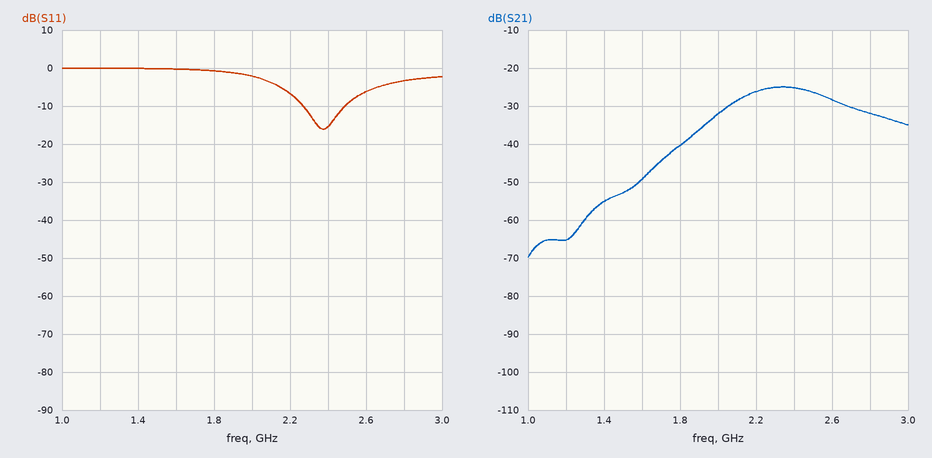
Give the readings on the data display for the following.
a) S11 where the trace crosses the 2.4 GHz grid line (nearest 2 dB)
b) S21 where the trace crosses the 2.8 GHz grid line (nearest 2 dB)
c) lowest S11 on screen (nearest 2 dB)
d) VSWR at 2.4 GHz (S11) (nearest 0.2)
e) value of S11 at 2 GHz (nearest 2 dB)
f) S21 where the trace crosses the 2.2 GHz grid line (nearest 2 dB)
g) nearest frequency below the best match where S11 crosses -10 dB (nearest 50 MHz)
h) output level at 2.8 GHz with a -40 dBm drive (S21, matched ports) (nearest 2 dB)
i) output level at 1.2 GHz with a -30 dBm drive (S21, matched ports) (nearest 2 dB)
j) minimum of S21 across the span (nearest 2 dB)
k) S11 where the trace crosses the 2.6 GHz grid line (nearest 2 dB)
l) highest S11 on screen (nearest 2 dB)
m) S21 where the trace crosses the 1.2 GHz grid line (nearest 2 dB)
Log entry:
-16 dB
-32 dB
-16 dB
1.4
-2 dB
-26 dB
2.25 GHz
-72 dBm
-96 dBm
-70 dB
-6 dB
0 dB
-66 dB
